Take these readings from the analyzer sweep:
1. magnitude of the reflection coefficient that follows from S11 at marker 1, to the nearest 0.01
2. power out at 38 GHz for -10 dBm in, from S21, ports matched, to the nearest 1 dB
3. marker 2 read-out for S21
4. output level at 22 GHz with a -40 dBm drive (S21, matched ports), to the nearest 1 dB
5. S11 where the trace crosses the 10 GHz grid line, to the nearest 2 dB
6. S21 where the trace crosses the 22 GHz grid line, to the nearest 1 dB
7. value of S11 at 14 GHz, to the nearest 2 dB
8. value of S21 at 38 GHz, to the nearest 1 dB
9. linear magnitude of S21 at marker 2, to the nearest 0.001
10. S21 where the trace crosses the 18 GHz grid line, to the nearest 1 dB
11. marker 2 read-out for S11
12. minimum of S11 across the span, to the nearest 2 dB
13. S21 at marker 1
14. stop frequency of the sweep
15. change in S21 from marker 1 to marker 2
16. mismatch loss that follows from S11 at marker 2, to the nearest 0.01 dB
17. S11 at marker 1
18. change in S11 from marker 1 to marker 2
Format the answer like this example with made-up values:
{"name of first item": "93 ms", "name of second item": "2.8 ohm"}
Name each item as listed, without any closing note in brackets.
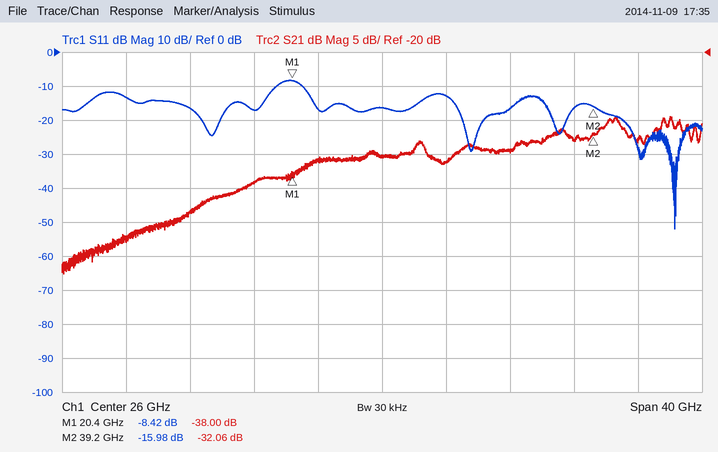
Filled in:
{"magnitude of the reflection coefficient that follows from S11 at marker 1, to the nearest 0.01": "0.38", "power out at 38 GHz for -10 dBm in, from S21, ports matched, to the nearest 1 dB": "-43 dBm", "marker 2 read-out for S21": "-32.06 dB", "output level at 22 GHz with a -40 dBm drive (S21, matched ports), to the nearest 1 dB": "-76 dBm", "S11 where the trace crosses the 10 GHz grid line, to the nearest 2 dB": "-14 dB", "S21 where the trace crosses the 22 GHz grid line, to the nearest 1 dB": "-36 dB", "value of S11 at 14 GHz, to the nearest 2 dB": "-16 dB", "value of S21 at 38 GHz, to the nearest 1 dB": "-33 dB", "linear magnitude of S21 at marker 2, to the nearest 0.001": "0.025", "S21 where the trace crosses the 18 GHz grid line, to the nearest 1 dB": "-39 dB", "marker 2 read-out for S11": "-15.98 dB", "minimum of S11 across the span, to the nearest 2 dB": "-52 dB", "S21 at marker 1": "-38.00 dB", "stop frequency of the sweep": "46 GHz", "change in S21 from marker 1 to marker 2": "5.94 dB", "mismatch loss that follows from S11 at marker 2, to the nearest 0.01 dB": "0.11 dB", "S11 at marker 1": "-8.42 dB", "change in S11 from marker 1 to marker 2": "-7.56 dB"}
